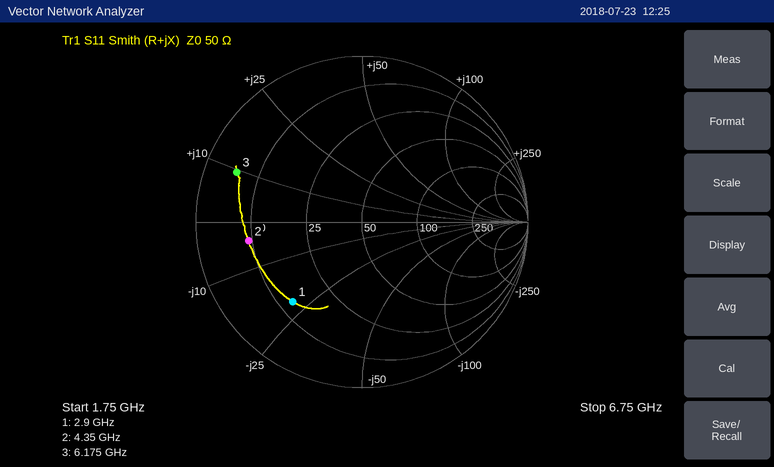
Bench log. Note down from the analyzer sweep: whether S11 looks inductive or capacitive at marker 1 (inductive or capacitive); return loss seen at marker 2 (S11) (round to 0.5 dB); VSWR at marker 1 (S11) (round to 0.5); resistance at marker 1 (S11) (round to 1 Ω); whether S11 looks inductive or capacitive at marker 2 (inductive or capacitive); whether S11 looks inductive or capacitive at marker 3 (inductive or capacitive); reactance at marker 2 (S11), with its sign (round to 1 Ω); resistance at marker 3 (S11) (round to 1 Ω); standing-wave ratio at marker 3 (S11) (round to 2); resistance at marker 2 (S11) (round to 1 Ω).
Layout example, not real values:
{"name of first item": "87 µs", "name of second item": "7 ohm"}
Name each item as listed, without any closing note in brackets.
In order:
{"whether S11 looks inductive or capacitive at marker 1": "capacitive", "return loss seen at marker 2 (S11)": "3.0 dB", "VSWR at marker 1 (S11)": "4.5", "resistance at marker 1 (S11)": "13 Ω", "whether S11 looks inductive or capacitive at marker 2": "capacitive", "whether S11 looks inductive or capacitive at marker 3": "inductive", "reactance at marker 2 (S11), with its sign": "-4 Ω", "resistance at marker 3 (S11)": "5 Ω", "standing-wave ratio at marker 3 (S11)": "10", "resistance at marker 2 (S11)": "9 Ω"}
